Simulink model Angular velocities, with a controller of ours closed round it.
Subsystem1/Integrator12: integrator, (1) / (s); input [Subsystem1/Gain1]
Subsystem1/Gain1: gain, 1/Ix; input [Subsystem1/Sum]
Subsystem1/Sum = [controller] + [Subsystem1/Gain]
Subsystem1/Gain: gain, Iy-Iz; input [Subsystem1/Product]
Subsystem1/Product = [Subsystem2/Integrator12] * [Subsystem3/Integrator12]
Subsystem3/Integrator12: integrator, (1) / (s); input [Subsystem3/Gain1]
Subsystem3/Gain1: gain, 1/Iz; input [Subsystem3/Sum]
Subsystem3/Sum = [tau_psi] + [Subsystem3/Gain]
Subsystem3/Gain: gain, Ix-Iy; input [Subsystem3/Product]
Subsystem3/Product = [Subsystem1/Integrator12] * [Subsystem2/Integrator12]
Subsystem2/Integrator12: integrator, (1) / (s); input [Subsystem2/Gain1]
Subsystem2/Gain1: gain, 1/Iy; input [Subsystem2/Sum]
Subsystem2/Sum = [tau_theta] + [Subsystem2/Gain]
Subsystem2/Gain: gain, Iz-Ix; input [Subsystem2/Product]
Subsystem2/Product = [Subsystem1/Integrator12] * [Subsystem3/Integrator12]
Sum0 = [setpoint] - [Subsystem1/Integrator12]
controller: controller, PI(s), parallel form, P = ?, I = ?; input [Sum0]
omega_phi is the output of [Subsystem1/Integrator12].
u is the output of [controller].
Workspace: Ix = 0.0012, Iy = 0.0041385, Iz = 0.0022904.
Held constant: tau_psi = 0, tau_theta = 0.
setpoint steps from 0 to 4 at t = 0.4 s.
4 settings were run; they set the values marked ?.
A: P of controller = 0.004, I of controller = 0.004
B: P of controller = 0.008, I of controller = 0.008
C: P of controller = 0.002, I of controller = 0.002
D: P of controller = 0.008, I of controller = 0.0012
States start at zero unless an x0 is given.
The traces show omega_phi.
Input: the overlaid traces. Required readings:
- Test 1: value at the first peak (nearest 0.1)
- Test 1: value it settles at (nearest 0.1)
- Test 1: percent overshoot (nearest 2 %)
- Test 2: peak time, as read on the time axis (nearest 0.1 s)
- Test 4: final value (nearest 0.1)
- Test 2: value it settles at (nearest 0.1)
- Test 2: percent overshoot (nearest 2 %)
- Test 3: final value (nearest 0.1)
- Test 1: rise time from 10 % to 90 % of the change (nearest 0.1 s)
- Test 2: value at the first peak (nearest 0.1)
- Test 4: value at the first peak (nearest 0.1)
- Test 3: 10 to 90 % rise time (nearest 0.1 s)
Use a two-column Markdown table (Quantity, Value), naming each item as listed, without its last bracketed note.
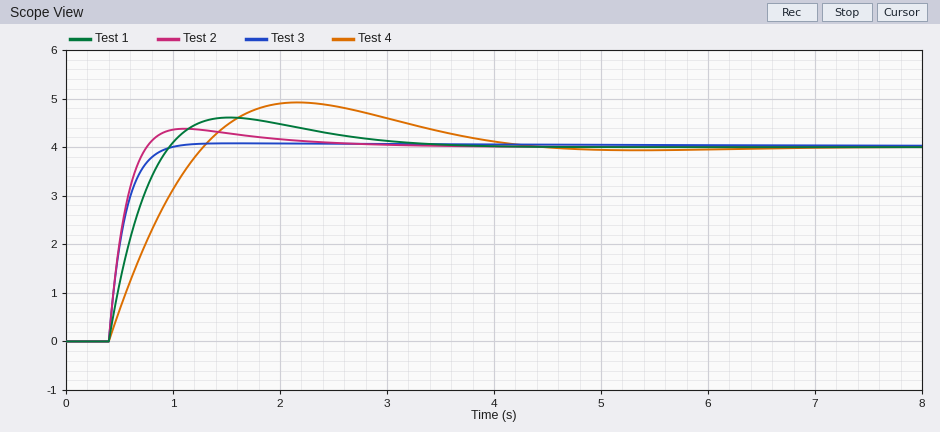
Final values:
| Quantity | Value |
|---|---|
| Test 1: value at the first peak | 4.6 |
| Test 1: value it settles at | 4.0 |
| Test 1: percent overshoot | 16 % |
| Test 2: peak time, as read on the time axis | 1.1 s |
| Test 4: final value | 4.0 |
| Test 2: value it settles at | 4.0 |
| Test 2: percent overshoot | 10 % |
| Test 3: final value | 4.0 |
| Test 1: rise time from 10 % to 90 % of the change | 0.4 s |
| Test 2: value at the first peak | 4.4 |
| Test 4: value at the first peak | 4.9 |
| Test 3: 10 to 90 % rise time | 0.3 s |
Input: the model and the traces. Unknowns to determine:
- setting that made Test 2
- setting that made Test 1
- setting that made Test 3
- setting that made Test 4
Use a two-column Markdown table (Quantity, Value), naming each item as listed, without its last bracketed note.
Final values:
| Quantity | Value |
|---|---|
| setting that made Test 2 | B |
| setting that made Test 1 | A |
| setting that made Test 3 | D |
| setting that made Test 4 | C |
